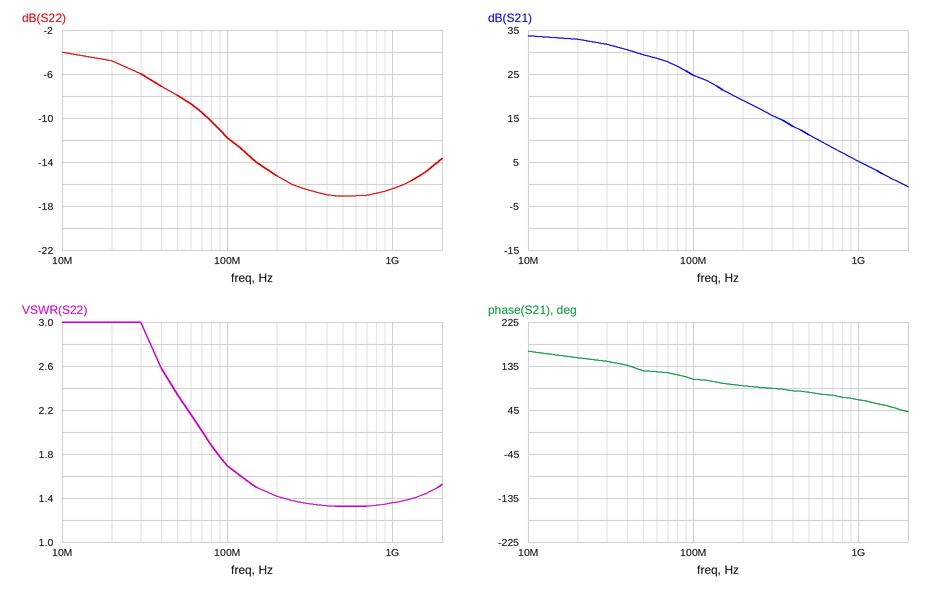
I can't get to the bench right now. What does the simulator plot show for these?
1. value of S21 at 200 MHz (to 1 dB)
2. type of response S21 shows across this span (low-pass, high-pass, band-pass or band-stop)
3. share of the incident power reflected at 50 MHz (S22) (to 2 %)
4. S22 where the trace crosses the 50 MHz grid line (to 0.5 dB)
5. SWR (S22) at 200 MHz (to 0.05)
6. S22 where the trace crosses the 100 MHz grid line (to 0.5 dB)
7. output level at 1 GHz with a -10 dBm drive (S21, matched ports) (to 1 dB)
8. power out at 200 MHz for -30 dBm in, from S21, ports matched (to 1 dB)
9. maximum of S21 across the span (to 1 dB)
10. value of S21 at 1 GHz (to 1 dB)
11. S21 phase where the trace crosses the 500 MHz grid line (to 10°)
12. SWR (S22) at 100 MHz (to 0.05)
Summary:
19 dB
low-pass
16 %
-8.0 dB
1.40
-12.0 dB
-5 dBm
-11 dBm
34 dB
5 dB
80°
1.70
